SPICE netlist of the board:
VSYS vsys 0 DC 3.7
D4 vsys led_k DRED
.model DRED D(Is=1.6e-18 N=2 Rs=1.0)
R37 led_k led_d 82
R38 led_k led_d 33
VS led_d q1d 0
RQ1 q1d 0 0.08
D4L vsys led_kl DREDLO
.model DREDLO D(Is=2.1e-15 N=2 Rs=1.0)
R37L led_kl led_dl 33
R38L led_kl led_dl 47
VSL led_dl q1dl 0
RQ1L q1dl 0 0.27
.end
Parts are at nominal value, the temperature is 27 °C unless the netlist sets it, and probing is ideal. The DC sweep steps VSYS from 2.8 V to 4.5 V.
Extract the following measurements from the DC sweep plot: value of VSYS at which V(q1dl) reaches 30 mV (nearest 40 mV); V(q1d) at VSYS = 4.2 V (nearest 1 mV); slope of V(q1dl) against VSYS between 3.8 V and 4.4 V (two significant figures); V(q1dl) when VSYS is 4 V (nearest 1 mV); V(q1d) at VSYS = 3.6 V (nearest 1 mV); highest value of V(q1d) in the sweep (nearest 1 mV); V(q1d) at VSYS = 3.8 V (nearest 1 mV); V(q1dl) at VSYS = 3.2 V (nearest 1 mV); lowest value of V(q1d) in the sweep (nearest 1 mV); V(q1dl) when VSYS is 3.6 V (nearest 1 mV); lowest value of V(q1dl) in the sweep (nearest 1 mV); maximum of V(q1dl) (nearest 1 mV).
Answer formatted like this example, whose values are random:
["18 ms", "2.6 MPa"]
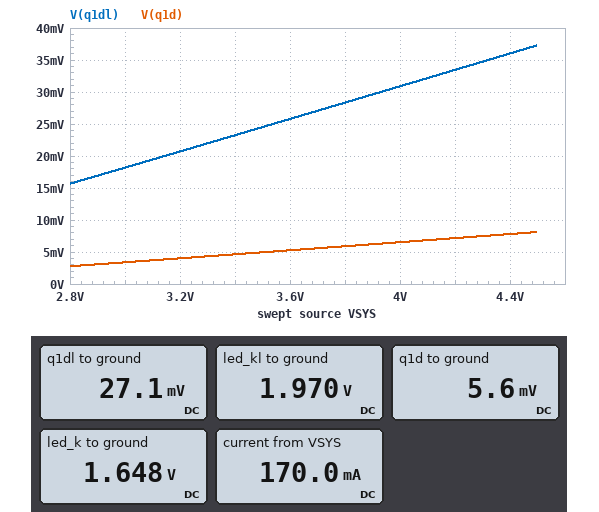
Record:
["3.92 V", "7 mV", "0.013 V/V", "31 mV", "5 mV", "8 mV", "6 mV", "21 mV", "3 mV", "26 mV", "16 mV", "37 mV"]
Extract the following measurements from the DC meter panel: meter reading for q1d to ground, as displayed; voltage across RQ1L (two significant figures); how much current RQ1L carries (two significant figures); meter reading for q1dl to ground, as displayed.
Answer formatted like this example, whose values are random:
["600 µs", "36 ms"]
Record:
["5.6 mV", "27 mV", "100 mA", "27.1 mV"]
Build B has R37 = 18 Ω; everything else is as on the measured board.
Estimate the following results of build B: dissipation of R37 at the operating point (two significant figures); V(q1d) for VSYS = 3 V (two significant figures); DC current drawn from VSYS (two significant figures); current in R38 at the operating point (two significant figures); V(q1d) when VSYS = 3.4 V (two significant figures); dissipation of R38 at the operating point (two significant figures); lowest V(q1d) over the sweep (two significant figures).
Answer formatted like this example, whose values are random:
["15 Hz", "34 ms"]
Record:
["130 mW", "6.4 mV", "230 mA", "47 mA", "8.8 mV", "72 mW", "5.2 mV"]
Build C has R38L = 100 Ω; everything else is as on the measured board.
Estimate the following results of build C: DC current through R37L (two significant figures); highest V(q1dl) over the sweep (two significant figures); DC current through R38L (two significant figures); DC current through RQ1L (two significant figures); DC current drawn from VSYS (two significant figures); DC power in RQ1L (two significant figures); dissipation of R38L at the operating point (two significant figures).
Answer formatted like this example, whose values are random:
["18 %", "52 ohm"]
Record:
["60 mA", "30 mV", "20 mA", "80 mA", "150 mA", "1.7 mW", "39 mW"]
